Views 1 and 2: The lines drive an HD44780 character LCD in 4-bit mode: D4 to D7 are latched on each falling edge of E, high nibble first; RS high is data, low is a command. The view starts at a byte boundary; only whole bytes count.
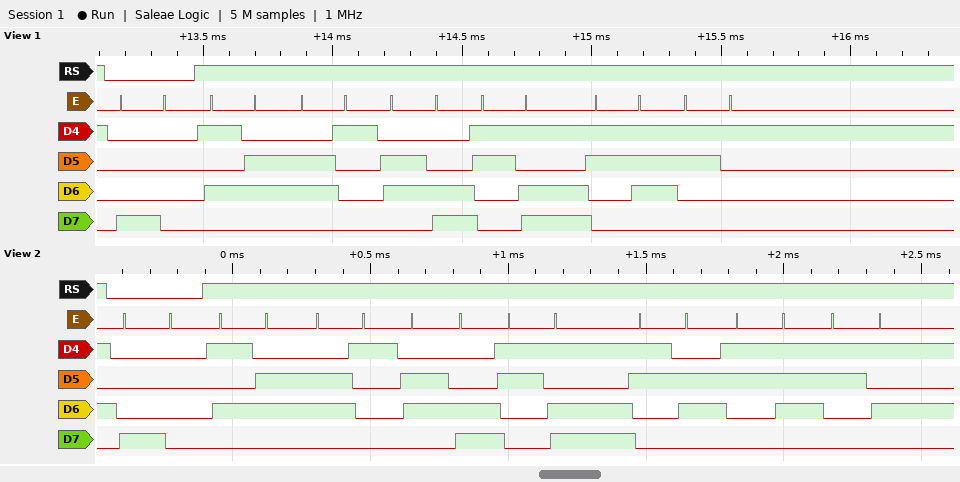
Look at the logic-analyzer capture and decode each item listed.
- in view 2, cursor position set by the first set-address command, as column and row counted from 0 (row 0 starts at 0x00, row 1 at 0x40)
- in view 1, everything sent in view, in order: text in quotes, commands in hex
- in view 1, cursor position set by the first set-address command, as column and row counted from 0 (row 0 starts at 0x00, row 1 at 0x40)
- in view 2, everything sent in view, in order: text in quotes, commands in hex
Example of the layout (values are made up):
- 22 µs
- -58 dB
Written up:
- column 0, row 0
- 0x80 "Val=71"
- column 0, row 0
- 0x80 "Val=675"
